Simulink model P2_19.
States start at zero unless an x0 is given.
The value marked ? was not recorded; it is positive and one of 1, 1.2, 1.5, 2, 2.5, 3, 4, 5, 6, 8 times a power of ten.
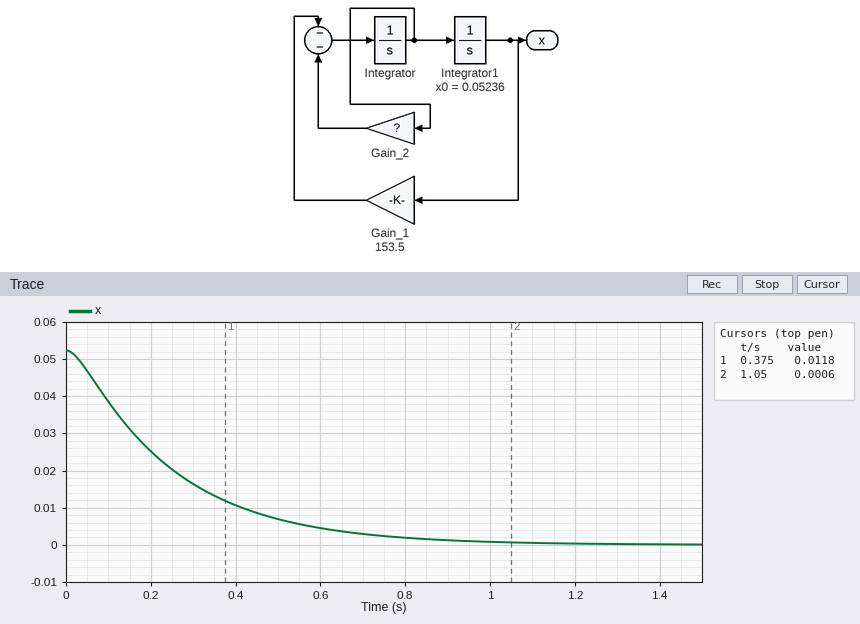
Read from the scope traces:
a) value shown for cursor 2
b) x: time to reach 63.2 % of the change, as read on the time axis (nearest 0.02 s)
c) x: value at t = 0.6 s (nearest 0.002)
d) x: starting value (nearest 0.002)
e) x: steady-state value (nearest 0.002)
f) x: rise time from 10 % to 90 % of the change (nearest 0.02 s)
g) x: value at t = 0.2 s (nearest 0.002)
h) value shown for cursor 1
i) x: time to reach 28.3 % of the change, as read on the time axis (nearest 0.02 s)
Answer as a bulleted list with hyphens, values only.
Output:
- 0.0006
- 0.26 s
- 0.004
- 0.052
- 0.000
- 0.52 s
- 0.026
- 0.0118
- 0.10 s
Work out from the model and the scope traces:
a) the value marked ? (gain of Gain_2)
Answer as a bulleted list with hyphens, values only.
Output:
- 40
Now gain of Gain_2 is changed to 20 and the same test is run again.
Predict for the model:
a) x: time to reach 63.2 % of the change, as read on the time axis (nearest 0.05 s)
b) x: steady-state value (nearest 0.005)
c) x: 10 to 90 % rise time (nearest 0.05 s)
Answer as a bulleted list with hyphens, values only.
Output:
- 0.15 s
- 0.000
- 0.20 s
